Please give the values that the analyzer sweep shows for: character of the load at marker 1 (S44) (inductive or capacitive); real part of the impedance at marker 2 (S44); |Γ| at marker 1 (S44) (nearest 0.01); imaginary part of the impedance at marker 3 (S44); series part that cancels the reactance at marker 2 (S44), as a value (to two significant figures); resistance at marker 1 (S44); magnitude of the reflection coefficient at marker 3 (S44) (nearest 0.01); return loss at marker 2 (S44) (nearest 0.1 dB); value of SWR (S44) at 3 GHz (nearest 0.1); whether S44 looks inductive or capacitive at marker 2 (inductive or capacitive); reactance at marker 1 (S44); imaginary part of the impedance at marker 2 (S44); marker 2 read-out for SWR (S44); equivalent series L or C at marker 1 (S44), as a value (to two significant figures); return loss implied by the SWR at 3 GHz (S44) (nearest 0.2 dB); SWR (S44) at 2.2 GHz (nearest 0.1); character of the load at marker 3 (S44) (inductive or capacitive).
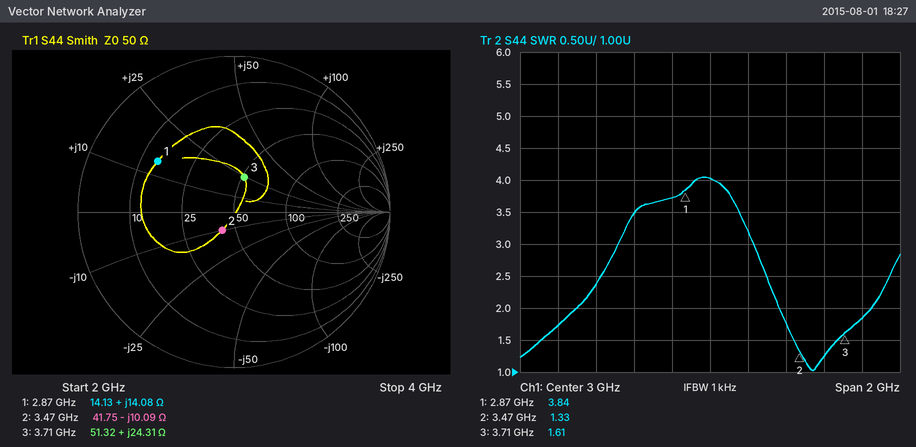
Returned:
inductive
41.75 Ω
0.59
+24.31 Ω
460 pH
14.13 Ω
0.23
17.0 dB
4.0
capacitive
+14.08 Ω
-10.09 Ω
1.33
780 pH
4.4 dB
1.7
inductive
